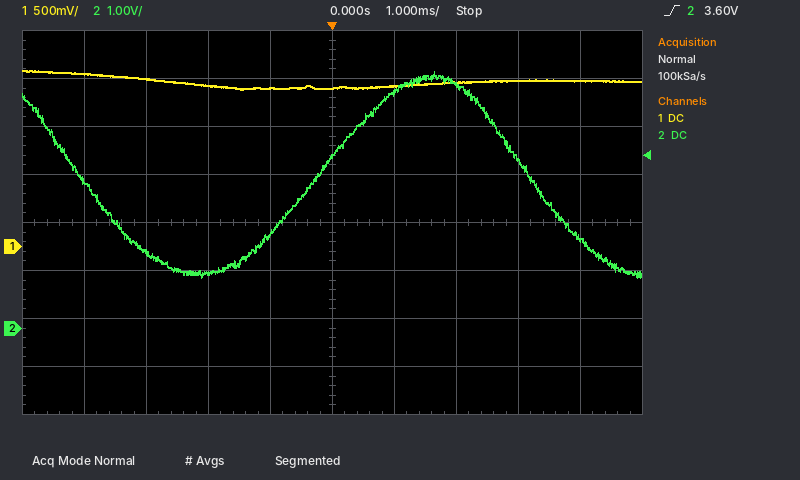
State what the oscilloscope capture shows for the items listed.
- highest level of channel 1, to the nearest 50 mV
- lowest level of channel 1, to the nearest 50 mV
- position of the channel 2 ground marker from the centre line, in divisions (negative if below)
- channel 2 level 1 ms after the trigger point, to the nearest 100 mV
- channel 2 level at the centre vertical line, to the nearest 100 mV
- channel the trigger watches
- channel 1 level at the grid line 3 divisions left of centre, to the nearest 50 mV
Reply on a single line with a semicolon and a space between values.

1.85 V; 1.65 V; -2.2 div; 4.9 V; 3.6 V; channel 2; 1.75 V
